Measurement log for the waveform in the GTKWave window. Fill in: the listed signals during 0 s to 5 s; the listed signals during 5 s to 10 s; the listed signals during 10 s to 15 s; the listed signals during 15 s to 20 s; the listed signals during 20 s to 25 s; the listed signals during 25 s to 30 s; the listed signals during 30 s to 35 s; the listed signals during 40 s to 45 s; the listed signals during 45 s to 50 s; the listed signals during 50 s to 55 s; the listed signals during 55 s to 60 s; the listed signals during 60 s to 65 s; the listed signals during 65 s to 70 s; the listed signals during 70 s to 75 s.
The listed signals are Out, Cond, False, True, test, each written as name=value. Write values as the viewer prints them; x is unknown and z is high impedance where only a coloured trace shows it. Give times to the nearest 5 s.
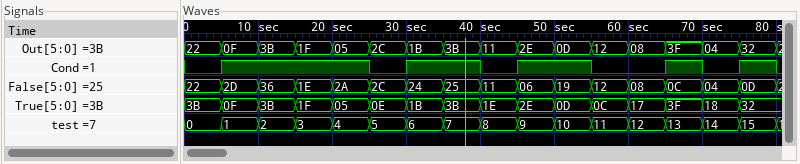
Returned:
Out=22, Cond=0, False=22, True=3B, test=0
Out=0F, Cond=1, False=2D, True=0F, test=1
Out=3B, Cond=1, False=36, True=3B, test=2
Out=1F, Cond=1, False=1E, True=1F, test=3
Out=05, Cond=1, False=2A, True=05, test=4
Out=2C, Cond=0, False=2C, True=0E, test=5
Out=1B, Cond=1, False=24, True=1B, test=6
Out=11, Cond=0, False=11, True=1E, test=8
Out=2E, Cond=1, False=06, True=2E, test=9
Out=0D, Cond=1, False=19, True=0D, test=10
Out=12, Cond=0, False=12, True=0C, test=11
Out=08, Cond=0, False=08, True=17, test=12
Out=3F, Cond=1, False=0C, True=3F, test=13
Out=04, Cond=0, False=04, True=18, test=14
